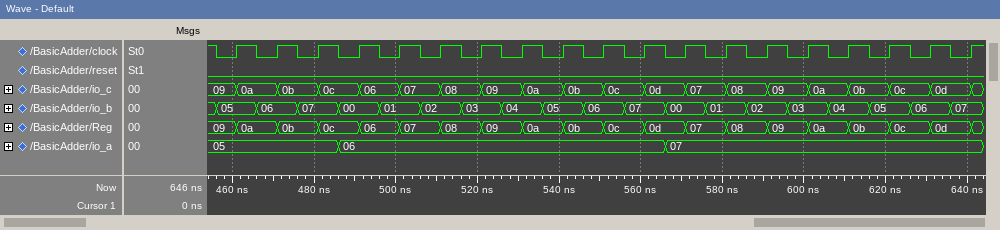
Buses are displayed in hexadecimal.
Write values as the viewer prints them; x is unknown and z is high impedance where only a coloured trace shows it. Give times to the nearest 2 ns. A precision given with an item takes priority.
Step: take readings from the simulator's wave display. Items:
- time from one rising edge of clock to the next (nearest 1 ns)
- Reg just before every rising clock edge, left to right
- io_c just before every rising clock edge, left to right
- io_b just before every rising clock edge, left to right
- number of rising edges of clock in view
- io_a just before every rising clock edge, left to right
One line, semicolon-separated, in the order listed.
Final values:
10 ns; 09, 0a, 0b, 0c, 06, 07, 08, 09, 0a, 0b, 0c, 0d, 07, 08, 09, 0a, 0b, 0c, 0d; 09, 0a, 0b, 0c, 06, 07, 08, 09, 0a, 0b, 0c, 0d, 07, 08, 09, 0a, 0b, 0c, 0d; 05, 06, 07, 00, 01, 02, 03, 04, 05, 06, 07, 00, 01, 02, 03, 04, 05, 06, 07; 19; 05, 05, 05, 06, 06, 06, 06, 06, 06, 06, 06, 07, 07, 07, 07, 07, 07, 07, 07
